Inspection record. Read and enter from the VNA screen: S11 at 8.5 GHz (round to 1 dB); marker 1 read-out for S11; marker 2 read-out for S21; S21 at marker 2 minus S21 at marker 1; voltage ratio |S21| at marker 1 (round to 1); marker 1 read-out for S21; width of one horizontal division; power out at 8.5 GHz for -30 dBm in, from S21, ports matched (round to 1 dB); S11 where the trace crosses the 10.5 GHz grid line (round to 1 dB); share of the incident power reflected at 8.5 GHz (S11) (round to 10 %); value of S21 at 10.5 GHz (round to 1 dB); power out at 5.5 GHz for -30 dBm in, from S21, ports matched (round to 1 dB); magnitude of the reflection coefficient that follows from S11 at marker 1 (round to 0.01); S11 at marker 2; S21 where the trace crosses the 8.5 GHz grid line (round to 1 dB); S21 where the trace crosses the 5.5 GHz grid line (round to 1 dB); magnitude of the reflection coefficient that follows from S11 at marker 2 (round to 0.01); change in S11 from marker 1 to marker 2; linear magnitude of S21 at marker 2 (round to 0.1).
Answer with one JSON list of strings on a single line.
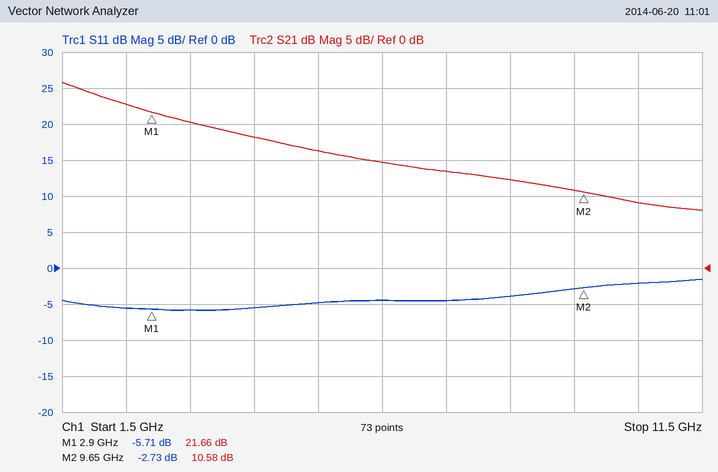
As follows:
["-4 dB", "-5.71 dB", "10.58 dB", "-11.08 dB", "12", "21.66 dB", "1 GHz", "-18 dBm", "-2 dB", "40 %", "9 dB", "-14 dBm", "0.52", "-2.73 dB", "12 dB", "16 dB", "0.73", "2.98 dB", "3.4"]
